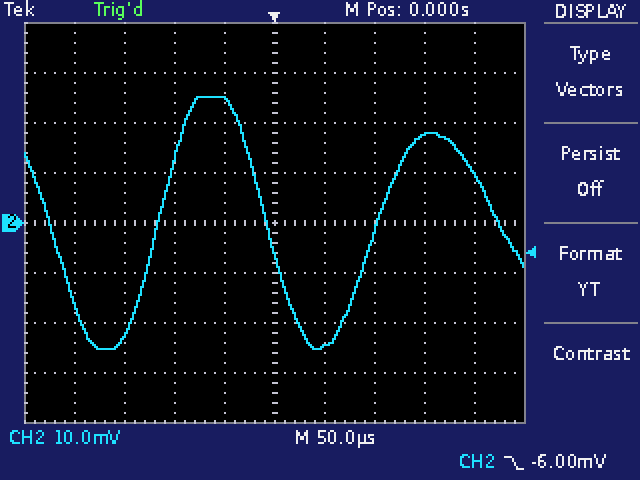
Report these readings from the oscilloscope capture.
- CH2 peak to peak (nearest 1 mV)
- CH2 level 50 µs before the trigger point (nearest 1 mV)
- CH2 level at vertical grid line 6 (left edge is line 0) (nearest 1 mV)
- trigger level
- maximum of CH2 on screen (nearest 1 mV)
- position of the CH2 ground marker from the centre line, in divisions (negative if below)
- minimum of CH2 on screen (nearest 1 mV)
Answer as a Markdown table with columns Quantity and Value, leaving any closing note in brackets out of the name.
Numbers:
| Quantity | Value |
|---|---|
| CH2 peak to peak | 50 mV |
| CH2 level 50 µs before the trigger point | 25 mV |
| CH2 level at vertical grid line 6 (left edge is line 0) | -25 mV |
| trigger level | -6.00 mV |
| maximum of CH2 on screen | 25 mV |
| position of the CH2 ground marker from the centre line, in divisions | 0.0 div |
| minimum of CH2 on screen | -25 mV |
